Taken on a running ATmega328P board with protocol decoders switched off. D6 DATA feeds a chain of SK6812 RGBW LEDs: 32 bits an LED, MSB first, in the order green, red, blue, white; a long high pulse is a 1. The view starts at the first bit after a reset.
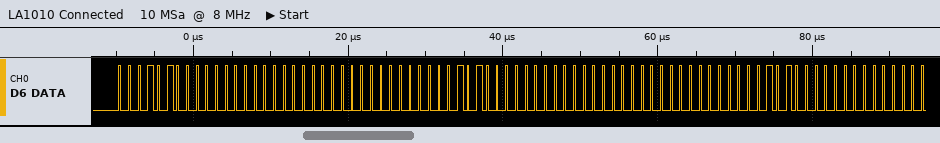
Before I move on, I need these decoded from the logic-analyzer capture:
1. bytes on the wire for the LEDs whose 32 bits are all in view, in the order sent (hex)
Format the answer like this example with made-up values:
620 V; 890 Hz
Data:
14 00 00 00 14 00 00 00
